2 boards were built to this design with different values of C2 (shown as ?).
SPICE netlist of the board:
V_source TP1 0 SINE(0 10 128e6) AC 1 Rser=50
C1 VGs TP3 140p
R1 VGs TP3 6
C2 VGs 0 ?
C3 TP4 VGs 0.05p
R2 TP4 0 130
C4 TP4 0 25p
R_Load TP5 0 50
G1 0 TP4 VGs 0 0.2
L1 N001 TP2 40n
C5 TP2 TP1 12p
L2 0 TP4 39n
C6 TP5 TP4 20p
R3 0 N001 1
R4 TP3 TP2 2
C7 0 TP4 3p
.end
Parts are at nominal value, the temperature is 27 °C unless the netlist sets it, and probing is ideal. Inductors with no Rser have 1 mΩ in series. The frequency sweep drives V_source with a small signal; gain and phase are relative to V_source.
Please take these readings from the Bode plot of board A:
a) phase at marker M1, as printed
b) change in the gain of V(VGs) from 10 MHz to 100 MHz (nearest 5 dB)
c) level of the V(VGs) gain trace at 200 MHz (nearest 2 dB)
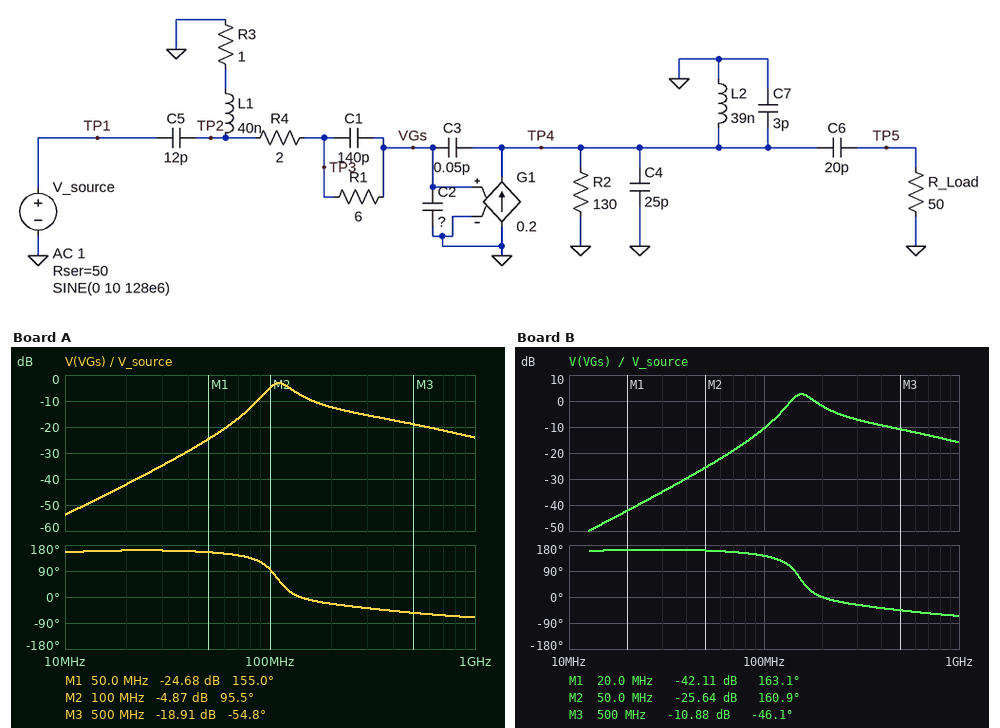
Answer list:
155.0 deg
50 dB
-12 dB
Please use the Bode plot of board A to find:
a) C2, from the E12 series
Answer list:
47 pF
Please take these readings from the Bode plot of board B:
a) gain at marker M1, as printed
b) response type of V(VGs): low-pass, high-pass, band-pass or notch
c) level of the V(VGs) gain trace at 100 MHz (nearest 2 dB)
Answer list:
-42.11 dB
band-pass
-10 dB
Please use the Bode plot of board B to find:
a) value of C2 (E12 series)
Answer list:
18 pF
